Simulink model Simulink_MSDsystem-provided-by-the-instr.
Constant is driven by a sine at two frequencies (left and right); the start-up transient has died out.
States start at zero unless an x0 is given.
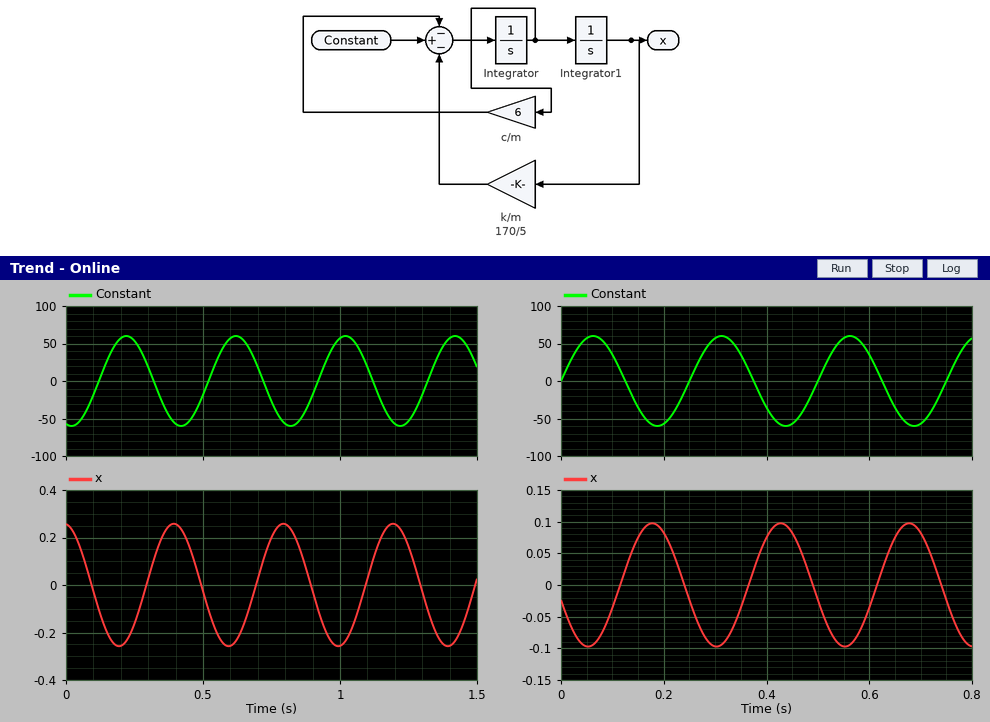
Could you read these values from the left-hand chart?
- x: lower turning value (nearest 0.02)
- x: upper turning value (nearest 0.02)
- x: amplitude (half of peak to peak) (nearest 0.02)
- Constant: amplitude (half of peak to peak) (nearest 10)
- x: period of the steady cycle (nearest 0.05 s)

-0.26
0.26
0.26
60
0.40 s
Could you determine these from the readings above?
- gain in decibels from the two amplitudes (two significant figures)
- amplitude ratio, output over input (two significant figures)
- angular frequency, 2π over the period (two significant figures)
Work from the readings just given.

-47 dB
0.0043
16 rad/s
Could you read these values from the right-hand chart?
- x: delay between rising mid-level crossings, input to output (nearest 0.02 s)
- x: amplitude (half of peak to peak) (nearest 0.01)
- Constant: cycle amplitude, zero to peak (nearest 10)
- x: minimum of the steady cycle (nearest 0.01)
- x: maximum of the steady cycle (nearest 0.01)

0.12 s
0.10
60
-0.10
0.10
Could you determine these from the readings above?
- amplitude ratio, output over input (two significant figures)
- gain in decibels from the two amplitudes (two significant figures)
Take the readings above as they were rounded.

0.0017
-56 dB
